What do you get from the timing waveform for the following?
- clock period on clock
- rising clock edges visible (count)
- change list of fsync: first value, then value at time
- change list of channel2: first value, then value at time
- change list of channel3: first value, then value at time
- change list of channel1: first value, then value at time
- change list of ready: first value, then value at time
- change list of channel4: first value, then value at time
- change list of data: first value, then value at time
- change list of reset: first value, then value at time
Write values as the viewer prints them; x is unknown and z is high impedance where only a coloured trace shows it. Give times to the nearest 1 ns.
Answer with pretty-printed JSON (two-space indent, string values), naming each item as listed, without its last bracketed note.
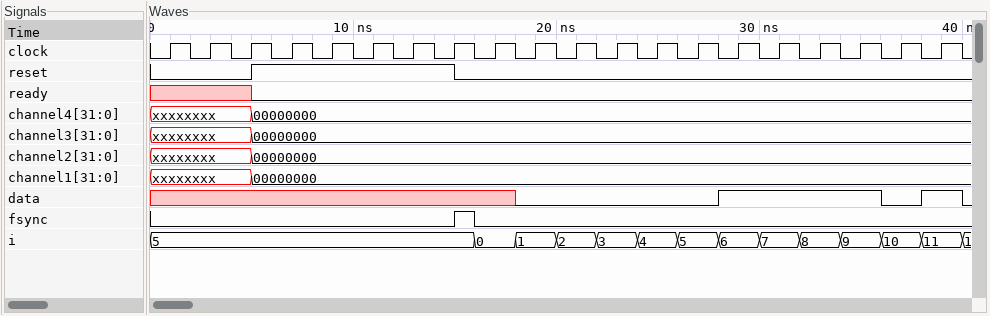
{
  "clock period on clock": "2 ns",
  "rising clock edges visible": "20",
  "change list of fsync: first value, then value at time": "0, 1 at 15 ns, 0 at 16 ns",
  "change list of channel2: first value, then value at time": "xxxxxxxx, 00000000 at 5 ns",
  "change list of channel3: first value, then value at time": "xxxxxxxx, 00000000 at 5 ns",
  "change list of channel1: first value, then value at time": "xxxxxxxx, 00000000 at 5 ns",
  "change list of ready: first value, then value at time": "x, 0 at 5 ns",
  "change list of channel4: first value, then value at time": "xxxxxxxx, 00000000 at 5 ns",
  "change list of data: first value, then value at time": "x, 0 at 18 ns, 1 at 28 ns, 0 at 36 ns, 1 at 38 ns, 0 at 40 ns",
  "change list of reset: first value, then value at time": "0, 1 at 5 ns, 0 at 15 ns"
}
